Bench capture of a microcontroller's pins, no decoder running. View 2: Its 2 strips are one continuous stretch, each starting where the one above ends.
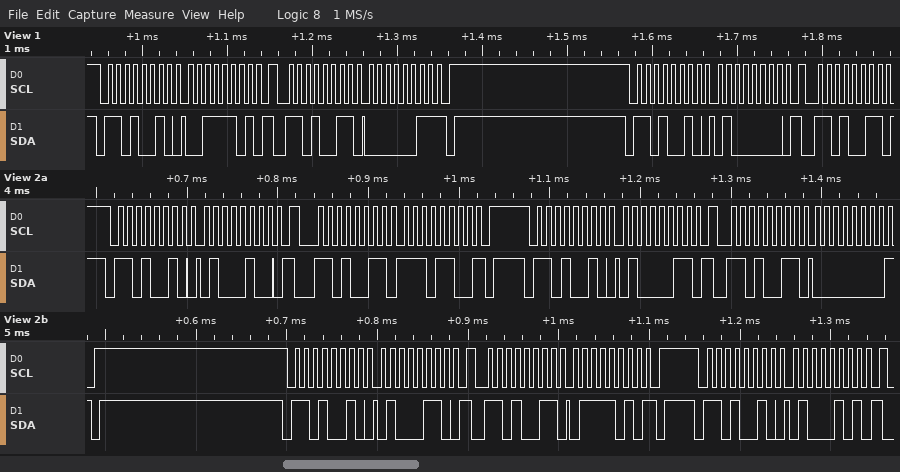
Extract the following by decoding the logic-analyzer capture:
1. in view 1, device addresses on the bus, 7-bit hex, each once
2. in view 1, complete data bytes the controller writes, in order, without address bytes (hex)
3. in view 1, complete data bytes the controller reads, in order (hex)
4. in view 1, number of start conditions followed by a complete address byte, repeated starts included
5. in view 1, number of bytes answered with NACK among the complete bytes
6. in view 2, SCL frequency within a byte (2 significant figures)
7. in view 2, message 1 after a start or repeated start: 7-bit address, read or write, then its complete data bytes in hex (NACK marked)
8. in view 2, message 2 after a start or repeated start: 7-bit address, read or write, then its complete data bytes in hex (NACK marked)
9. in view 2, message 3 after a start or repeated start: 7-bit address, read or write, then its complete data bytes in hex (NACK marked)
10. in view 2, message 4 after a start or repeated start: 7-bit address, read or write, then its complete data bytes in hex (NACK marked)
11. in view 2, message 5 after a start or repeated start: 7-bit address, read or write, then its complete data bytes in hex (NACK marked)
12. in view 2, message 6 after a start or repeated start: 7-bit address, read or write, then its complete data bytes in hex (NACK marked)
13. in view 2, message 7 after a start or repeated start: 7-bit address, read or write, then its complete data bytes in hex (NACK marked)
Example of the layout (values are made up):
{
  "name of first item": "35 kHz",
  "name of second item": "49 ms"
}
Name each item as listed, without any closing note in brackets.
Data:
{
  "in view 1, device addresses on the bus, 7-bit hex, each once": "0x69",
  "in view 1, complete data bytes the controller writes, in order, without address bytes": "3D 40",
  "in view 1, complete data bytes the controller reads, in order": "03",
  "in view 1, number of start conditions followed by a complete address byte, repeated starts included": "4",
  "in view 1, number of bytes answered with NACK among the complete bytes": "1",
  "in view 2, SCL frequency within a byte": "100 kHz",
  "in view 2, message 1 after a start or repeated start: 7-bit address, read or write, then its complete data bytes in hex": "0x69 write: 44",
  "in view 2, message 2 after a start or repeated start: 7-bit address, read or write, then its complete data bytes in hex": "0x69 read: EC NACK",
  "in view 2, message 3 after a start or repeated start: 7-bit address, read or write, then its complete data bytes in hex": "0x69 write: 43",
  "in view 2, message 4 after a start or repeated start: 7-bit address, read or write, then its complete data bytes in hex": "0x69 read: 00 NACK",
  "in view 2, message 5 after a start or repeated start: 7-bit address, read or write, then its complete data bytes in hex": "0x69 write: 46",
  "in view 2, message 6 after a start or repeated start: 7-bit address, read or write, then its complete data bytes in hex": "0x69 read: 7A NACK",
  "in view 2, message 7 after a start or repeated start: 7-bit address, read or write, then its complete data bytes in hex": "0x69 write: 45"
}
